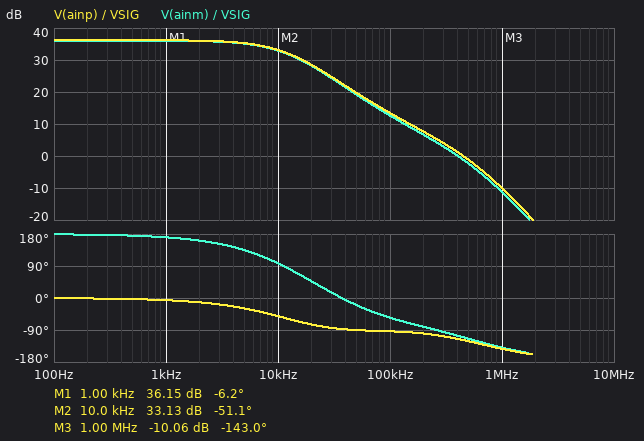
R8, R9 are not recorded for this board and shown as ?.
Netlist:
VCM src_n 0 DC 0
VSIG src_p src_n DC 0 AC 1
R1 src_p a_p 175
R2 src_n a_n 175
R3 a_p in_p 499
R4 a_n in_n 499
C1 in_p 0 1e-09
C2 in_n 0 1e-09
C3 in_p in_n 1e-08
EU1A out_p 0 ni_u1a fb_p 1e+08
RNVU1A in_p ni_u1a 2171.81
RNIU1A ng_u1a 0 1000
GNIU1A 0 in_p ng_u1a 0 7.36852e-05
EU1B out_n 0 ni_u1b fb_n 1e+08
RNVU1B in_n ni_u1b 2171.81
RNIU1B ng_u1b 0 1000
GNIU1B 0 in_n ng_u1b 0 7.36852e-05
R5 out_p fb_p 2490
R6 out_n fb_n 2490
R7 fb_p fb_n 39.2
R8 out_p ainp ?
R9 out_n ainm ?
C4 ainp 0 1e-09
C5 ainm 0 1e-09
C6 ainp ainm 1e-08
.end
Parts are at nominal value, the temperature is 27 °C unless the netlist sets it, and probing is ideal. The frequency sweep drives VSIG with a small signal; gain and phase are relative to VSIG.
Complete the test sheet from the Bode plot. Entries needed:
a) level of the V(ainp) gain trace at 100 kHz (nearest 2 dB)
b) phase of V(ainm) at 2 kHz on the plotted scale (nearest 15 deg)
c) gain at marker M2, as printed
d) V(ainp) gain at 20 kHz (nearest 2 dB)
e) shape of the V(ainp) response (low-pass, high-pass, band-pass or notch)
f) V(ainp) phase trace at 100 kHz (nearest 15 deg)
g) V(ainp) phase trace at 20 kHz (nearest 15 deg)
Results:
14 dB
165 deg
33.13 dB
28 dB
low-pass
-90 deg
-75 deg
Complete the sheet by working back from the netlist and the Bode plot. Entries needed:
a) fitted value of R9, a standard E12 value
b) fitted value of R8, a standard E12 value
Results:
560 Ω
150 Ω
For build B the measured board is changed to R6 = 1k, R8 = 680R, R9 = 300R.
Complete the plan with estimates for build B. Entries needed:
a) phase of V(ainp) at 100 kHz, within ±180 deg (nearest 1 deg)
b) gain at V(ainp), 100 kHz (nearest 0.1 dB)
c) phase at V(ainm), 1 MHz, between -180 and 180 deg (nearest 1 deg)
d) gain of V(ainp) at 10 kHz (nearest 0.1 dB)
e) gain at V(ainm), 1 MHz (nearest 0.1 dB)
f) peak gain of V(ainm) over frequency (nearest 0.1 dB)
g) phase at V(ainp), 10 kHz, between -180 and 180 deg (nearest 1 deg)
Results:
-138 deg
-0.5 dB
-143 deg
32.1 dB
-27.7 dB
28.1 dB
-74 deg
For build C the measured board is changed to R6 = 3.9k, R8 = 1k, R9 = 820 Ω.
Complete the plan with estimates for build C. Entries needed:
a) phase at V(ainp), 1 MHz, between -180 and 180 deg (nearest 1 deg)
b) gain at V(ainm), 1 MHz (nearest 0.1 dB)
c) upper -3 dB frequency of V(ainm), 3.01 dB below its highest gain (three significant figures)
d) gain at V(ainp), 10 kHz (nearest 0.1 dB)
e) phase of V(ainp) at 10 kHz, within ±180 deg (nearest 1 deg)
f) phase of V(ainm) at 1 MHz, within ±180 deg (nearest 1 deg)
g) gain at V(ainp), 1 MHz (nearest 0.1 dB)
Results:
4 deg
-28.0 dB
6.40 kHz
30.3 dB
-117 deg
3 deg
-32.4 dB
